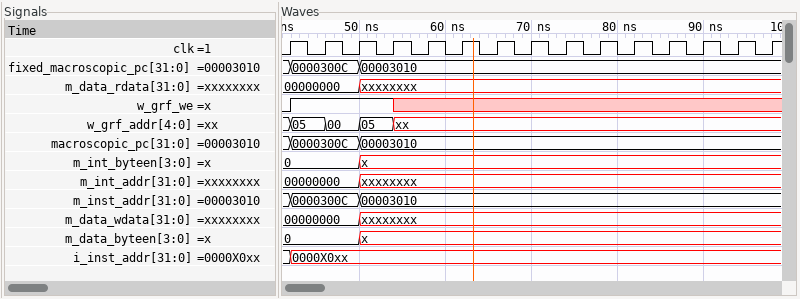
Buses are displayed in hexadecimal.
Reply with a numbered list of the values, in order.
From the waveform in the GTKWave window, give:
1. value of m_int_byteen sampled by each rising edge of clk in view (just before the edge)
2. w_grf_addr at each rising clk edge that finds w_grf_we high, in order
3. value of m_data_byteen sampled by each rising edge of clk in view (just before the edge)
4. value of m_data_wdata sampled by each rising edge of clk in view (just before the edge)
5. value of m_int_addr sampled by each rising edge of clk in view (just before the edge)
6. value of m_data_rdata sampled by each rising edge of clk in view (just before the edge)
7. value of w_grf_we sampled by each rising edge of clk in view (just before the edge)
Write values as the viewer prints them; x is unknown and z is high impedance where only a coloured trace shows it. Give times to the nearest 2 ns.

1. 0, 0, 0, x, x, x, x, x, x, x, x, x, x, x, x
2. 05, 00, 05
3. 0, 0, 0, x, x, x, x, x, x, x, x, x, x, x, x
4. 00000000, 00000000, 00000000, xxxxxxxx, xxxxxxxx, xxxxxxxx, xxxxxxxx, xxxxxxxx, xxxxxxxx, xxxxxxxx, xxxxxxxx, xxxxxxxx, xxxxxxxx, xxxxxxxx, xxxxxxxx
5. 00000000, 00000000, 00000000, xxxxxxxx, xxxxxxxx, xxxxxxxx, xxxxxxxx, xxxxxxxx, xxxxxxxx, xxxxxxxx, xxxxxxxx, xxxxxxxx, xxxxxxxx, xxxxxxxx, xxxxxxxx
6. 00000000, 00000000, 00000000, xxxxxxxx, xxxxxxxx, xxxxxxxx, xxxxxxxx, xxxxxxxx, xxxxxxxx, xxxxxxxx, xxxxxxxx, xxxxxxxx, xxxxxxxx, xxxxxxxx, xxxxxxxx
7. 0 1 1 1 x x x x x x x x x x x
